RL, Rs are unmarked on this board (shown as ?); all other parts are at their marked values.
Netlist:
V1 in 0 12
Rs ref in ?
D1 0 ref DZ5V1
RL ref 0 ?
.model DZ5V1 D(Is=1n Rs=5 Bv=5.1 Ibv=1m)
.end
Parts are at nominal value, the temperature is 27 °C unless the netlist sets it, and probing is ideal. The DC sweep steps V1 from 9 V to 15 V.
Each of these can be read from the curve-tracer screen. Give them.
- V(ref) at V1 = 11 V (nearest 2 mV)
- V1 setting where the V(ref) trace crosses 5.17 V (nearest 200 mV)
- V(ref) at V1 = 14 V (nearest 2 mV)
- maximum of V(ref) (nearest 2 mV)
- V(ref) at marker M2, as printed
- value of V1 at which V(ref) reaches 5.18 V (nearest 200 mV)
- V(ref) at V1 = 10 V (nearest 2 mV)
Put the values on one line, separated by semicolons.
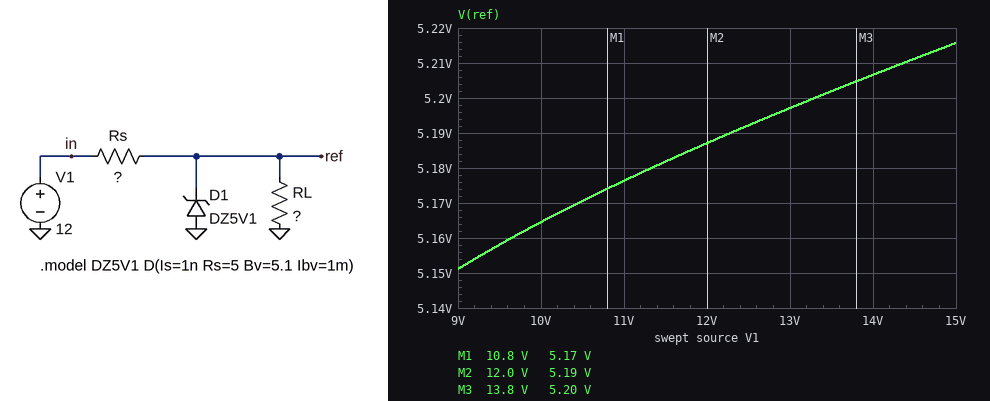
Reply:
5.176 V; 10.4 V; 5.206 V; 5.216 V; 5.19 V; 11.4 V; 5.164 V
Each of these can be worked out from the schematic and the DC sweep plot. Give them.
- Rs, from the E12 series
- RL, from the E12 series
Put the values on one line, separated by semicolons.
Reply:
820 Ω; 4.7 kΩ
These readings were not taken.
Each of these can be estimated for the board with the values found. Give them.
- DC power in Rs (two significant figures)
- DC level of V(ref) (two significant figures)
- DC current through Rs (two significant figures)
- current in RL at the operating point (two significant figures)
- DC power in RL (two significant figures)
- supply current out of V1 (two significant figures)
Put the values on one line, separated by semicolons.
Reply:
57 mW; 5.2 V; 8.3 mA; 1.1 mA; 5.7 mW; 8.3 mA
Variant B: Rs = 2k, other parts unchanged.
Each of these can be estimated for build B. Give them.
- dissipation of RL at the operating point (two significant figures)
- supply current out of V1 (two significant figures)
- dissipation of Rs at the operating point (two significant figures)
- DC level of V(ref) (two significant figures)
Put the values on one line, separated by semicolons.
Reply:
5.6 mW; 3.4 mA; 24 mW; 5.1 V
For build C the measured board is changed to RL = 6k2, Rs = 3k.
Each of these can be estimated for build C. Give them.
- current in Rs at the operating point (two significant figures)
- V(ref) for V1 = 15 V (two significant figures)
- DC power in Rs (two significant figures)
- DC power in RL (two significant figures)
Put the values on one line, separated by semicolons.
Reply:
2.3 mA; 5.1 V; 16 mW; 4.2 mW
